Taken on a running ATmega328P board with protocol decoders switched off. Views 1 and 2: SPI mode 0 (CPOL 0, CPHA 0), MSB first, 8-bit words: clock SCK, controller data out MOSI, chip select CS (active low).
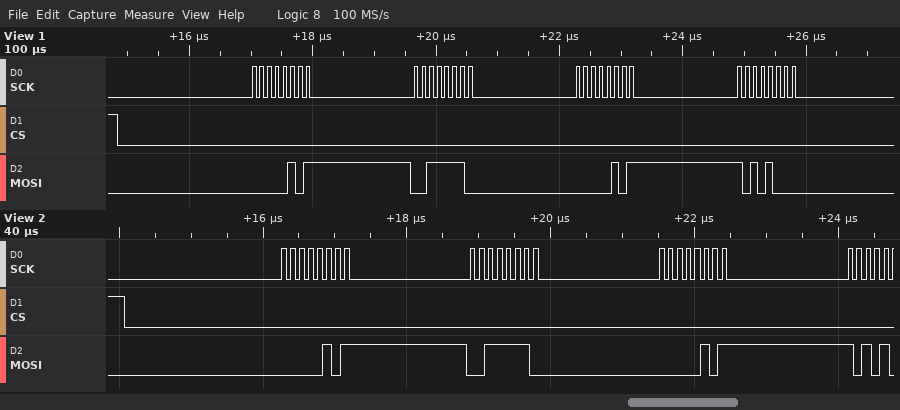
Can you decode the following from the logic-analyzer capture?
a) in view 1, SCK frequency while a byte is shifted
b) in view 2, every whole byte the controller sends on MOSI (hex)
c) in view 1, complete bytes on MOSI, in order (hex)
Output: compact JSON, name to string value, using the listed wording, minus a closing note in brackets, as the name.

{"in view 1, SCK frequency while a byte is shifted": "8 MHz", "in view 2, every whole byte the controller sends on MOSI": "05 3E 05", "in view 1, complete bytes on MOSI, in order": "05 3E 05 A8"}
